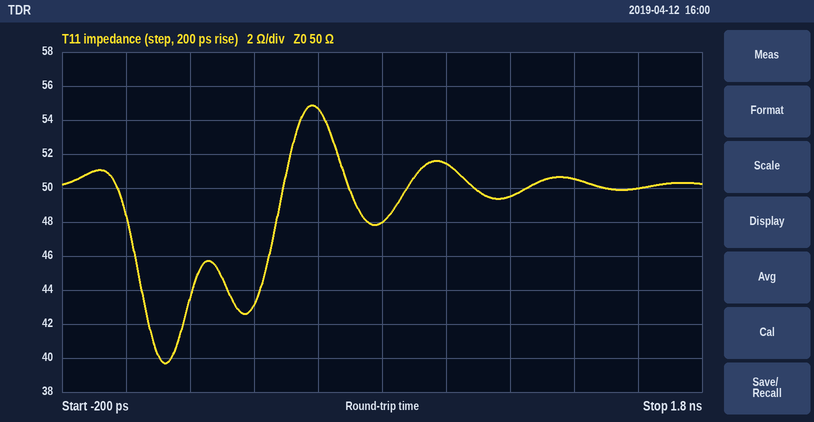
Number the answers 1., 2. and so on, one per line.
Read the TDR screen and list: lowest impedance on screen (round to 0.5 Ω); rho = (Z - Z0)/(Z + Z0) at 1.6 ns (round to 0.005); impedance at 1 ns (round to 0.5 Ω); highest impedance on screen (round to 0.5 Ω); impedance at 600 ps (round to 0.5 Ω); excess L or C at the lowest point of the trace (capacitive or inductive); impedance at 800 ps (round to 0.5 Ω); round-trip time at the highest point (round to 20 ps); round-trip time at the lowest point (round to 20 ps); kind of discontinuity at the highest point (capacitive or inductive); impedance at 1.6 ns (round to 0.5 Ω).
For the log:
1. 39.5 Ω
2. 0.000
3. 51.5 Ω
4. 55.0 Ω
5. 54.5 Ω
6. capacitive
7. 48.0 Ω
8. 580 ps
9. 120 ps
10. inductive
11. 50.0 Ω
